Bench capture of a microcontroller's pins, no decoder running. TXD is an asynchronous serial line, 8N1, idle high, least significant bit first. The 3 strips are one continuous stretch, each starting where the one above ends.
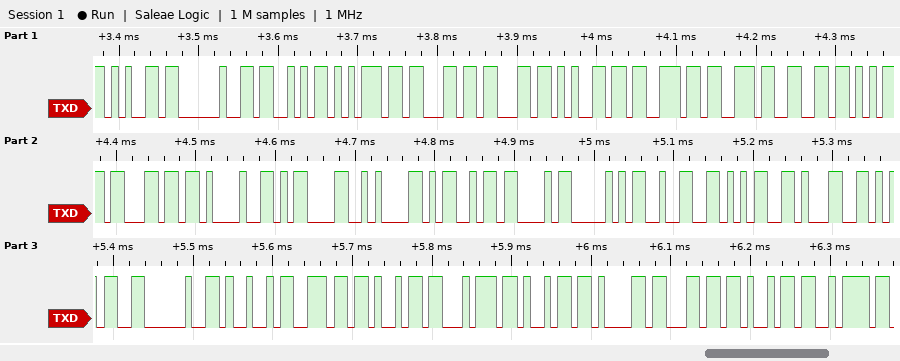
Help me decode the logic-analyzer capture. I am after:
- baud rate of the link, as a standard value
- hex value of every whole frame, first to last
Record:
115200 baud
65 20 53 75 63 63 65 73 73 66 75 6C 21 0D 0A 4D 43 50 32 35 31 35 20 49 6E 69 74 69 61 6C 69 7A
